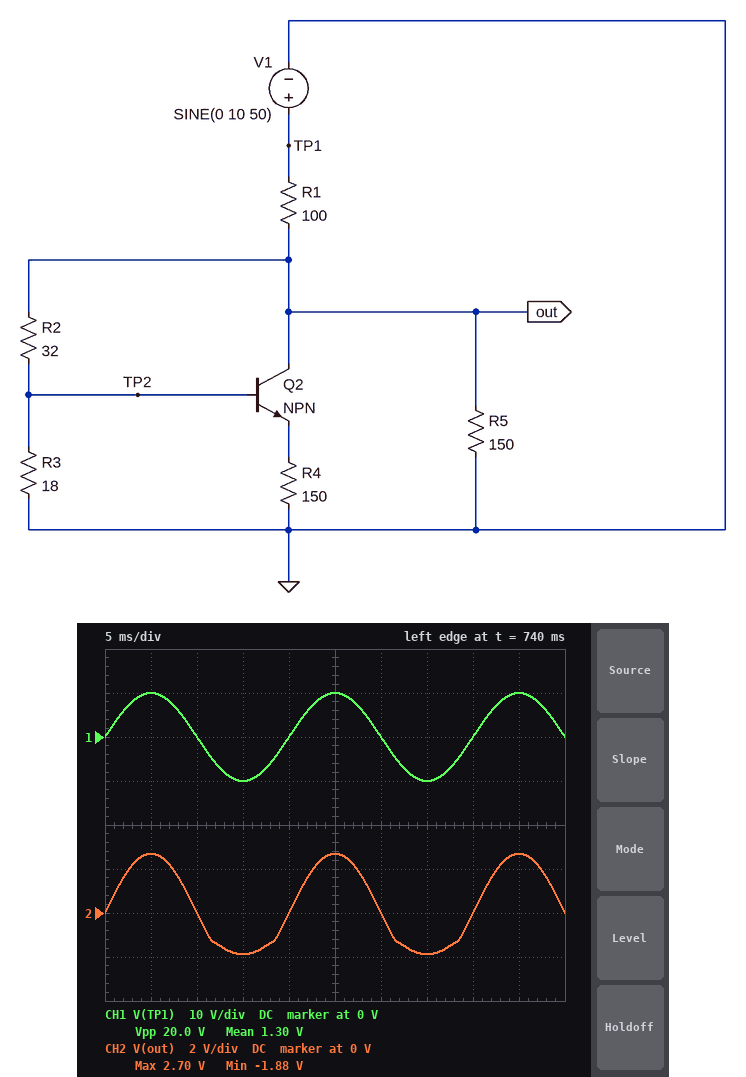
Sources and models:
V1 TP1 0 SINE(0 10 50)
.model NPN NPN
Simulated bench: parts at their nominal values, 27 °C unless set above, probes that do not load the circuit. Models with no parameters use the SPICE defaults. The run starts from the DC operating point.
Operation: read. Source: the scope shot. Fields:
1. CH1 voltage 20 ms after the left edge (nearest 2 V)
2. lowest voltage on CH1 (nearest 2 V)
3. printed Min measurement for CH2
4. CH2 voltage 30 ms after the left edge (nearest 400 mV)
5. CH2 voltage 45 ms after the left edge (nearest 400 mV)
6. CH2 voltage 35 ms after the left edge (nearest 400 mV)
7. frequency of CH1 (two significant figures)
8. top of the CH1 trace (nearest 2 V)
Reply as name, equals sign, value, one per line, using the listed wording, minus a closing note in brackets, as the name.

CH1 voltage 20 ms after the left edge = 0 V
lowest voltage on CH1 = -10 V
printed Min measurement for CH2 = -1.88 V
CH2 voltage 30 ms after the left edge = 0 V
CH2 voltage 45 ms after the left edge = 2.8 V
CH2 voltage 35 ms after the left edge = -2.0 V
frequency of CH1 = 50 Hz
top of the CH1 trace = 10 V
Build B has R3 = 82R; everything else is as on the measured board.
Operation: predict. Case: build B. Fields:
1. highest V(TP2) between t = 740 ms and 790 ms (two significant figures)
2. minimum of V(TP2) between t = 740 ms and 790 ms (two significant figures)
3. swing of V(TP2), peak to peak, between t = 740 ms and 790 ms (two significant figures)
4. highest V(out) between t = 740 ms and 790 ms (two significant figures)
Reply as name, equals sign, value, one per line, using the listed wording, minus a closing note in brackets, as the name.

highest V(TP2) between t = 740 ms and 790 ms = 2.5 V
minimum of V(TP2) between t = 740 ms and 790 ms = -2.7 V
swing of V(TP2), peak to peak, between t = 740 ms and 790 ms = 5.2 V
highest V(out) between t = 740 ms and 790 ms = 3.5 V
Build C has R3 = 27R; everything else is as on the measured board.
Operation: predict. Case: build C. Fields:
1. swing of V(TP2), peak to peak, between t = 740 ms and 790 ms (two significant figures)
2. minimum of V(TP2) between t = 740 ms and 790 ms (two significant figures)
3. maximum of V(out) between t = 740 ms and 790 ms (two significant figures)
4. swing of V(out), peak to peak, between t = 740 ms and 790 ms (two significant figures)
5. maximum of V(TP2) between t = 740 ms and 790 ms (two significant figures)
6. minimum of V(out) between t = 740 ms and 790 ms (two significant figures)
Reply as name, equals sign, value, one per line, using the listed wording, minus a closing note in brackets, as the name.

swing of V(TP2), peak to peak, between t = 740 ms and 790 ms = 2.6 V
minimum of V(TP2) between t = 740 ms and 790 ms = -1.3 V
maximum of V(out) between t = 740 ms and 790 ms = 2.9 V
swing of V(out), peak to peak, between t = 740 ms and 790 ms = 5.1 V
maximum of V(TP2) between t = 740 ms and 790 ms = 1.3 V
minimum of V(out) between t = 740 ms and 790 ms = -2.2 V
